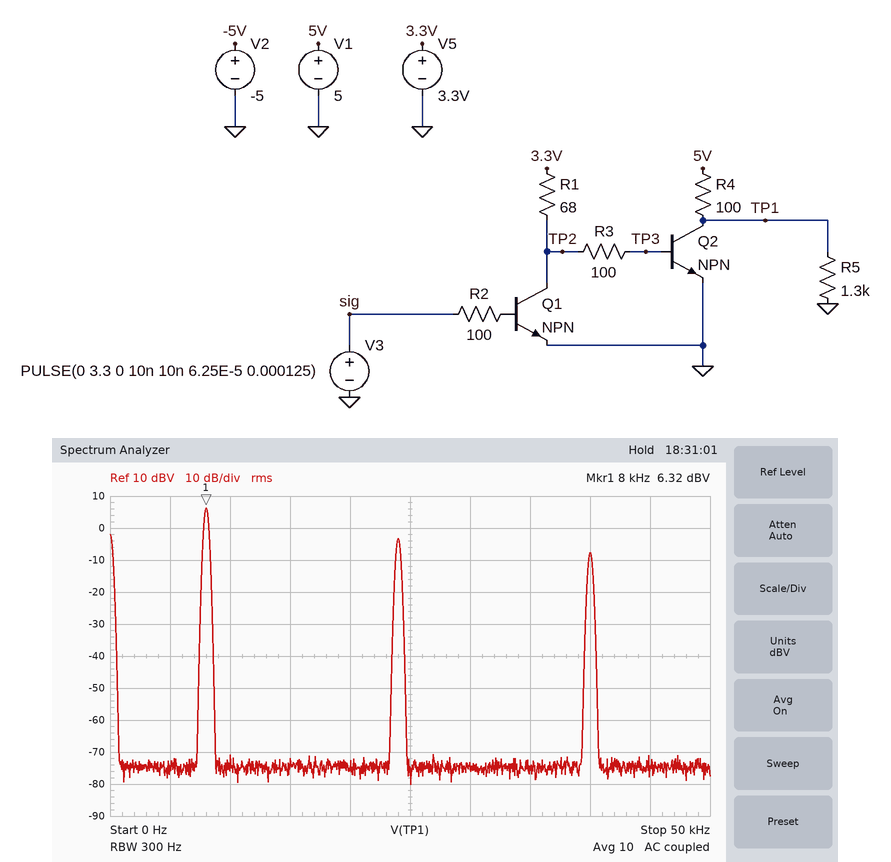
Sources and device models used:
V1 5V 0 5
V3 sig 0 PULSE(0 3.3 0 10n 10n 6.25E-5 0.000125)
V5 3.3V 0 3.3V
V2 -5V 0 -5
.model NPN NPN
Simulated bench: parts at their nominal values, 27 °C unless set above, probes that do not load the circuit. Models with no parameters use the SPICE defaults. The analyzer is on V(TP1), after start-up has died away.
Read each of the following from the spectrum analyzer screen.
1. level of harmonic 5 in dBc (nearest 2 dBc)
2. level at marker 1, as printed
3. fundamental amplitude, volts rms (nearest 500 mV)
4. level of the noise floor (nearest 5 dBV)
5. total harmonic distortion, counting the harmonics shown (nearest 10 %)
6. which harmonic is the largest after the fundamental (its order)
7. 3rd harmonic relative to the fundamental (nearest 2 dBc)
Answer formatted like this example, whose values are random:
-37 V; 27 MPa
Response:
-14 dBc; 6.32 dBV; 2.0 V; -75 dBV; 40 %; 3; -10 dBc
